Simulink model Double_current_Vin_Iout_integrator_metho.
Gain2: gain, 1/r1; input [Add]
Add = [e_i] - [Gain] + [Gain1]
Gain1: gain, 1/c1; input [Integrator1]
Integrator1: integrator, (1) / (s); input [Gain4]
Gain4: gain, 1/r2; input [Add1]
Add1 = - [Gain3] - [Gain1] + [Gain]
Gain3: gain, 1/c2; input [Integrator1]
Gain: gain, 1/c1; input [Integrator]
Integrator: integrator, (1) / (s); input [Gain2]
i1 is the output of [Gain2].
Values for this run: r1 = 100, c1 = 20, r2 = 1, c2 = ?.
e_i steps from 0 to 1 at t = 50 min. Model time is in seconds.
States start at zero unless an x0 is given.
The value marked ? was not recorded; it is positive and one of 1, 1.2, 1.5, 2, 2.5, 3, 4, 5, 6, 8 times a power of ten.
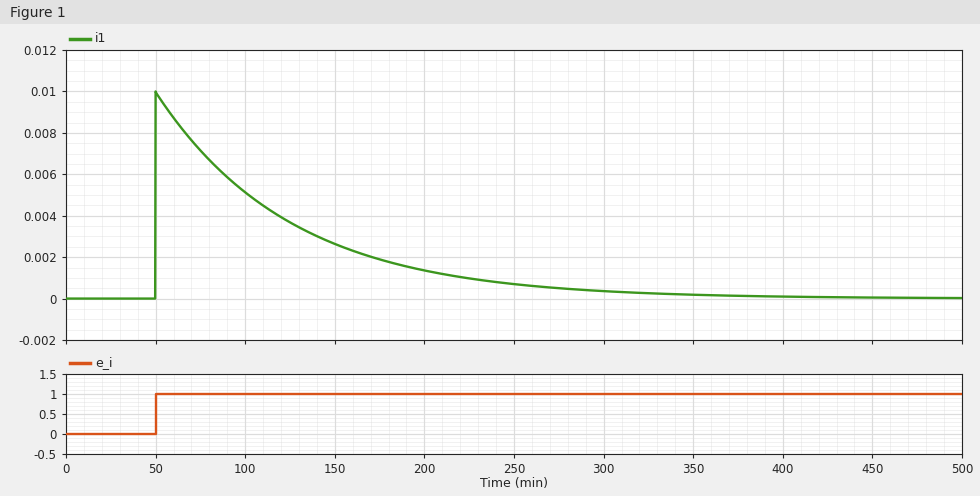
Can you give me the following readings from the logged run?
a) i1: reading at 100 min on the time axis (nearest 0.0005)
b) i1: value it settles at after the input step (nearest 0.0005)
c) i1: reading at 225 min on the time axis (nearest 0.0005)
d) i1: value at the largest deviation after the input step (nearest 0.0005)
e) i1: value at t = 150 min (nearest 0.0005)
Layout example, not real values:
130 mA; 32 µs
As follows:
0.0050; 0.0000; 0.0010; 0.0100; 0.0025
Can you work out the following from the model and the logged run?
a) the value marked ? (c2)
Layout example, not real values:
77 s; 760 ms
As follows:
25
